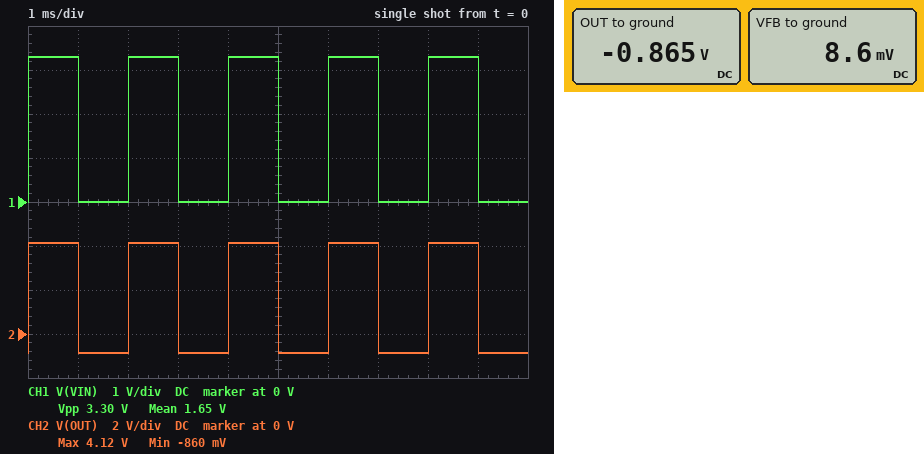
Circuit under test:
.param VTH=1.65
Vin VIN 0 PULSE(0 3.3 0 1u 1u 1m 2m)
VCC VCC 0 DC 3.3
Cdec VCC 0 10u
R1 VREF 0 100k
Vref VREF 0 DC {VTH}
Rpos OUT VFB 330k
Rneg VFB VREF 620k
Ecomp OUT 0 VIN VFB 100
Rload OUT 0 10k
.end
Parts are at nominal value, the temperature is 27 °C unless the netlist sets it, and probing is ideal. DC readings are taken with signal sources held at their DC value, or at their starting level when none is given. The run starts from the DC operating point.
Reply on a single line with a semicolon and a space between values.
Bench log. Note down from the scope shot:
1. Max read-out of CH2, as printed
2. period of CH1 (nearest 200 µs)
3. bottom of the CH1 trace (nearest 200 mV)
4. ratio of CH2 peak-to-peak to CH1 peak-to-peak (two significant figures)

4.12 V; 2.0 ms; 0 V; 1.5
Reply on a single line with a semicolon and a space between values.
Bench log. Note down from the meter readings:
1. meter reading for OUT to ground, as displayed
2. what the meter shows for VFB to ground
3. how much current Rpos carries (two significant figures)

-0.865 V; 8.6 mV; 2.6 µA
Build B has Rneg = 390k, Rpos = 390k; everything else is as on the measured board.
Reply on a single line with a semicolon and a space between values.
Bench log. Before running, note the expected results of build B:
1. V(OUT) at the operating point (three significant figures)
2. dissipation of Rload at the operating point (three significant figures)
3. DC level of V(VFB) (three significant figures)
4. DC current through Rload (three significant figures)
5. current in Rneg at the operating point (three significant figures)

-1.62 V; 262 µW; 16.2 mV; 162 µA; 4.19 µA
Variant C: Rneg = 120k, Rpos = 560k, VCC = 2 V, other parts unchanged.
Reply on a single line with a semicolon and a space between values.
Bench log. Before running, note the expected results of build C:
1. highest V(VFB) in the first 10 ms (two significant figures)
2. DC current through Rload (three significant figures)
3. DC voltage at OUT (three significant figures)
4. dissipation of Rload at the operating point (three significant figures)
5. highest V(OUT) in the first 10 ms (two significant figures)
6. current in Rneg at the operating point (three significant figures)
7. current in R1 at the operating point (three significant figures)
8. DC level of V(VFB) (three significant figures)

3.2 V; 729 µA; -7.29 V; 5.31 mW; 10 V; 13.1 µA; 16.5 µA; 72.9 mV
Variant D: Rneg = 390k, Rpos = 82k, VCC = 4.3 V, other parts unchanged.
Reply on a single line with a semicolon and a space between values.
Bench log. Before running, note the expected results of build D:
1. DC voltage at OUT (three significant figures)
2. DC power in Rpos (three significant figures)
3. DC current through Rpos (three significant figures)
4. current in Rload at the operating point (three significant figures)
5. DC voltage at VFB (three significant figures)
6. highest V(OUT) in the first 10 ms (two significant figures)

-343 mV; 1.46 µW; 4.22 µA; 34.3 µA; 3.43 mV; 3.6 V
